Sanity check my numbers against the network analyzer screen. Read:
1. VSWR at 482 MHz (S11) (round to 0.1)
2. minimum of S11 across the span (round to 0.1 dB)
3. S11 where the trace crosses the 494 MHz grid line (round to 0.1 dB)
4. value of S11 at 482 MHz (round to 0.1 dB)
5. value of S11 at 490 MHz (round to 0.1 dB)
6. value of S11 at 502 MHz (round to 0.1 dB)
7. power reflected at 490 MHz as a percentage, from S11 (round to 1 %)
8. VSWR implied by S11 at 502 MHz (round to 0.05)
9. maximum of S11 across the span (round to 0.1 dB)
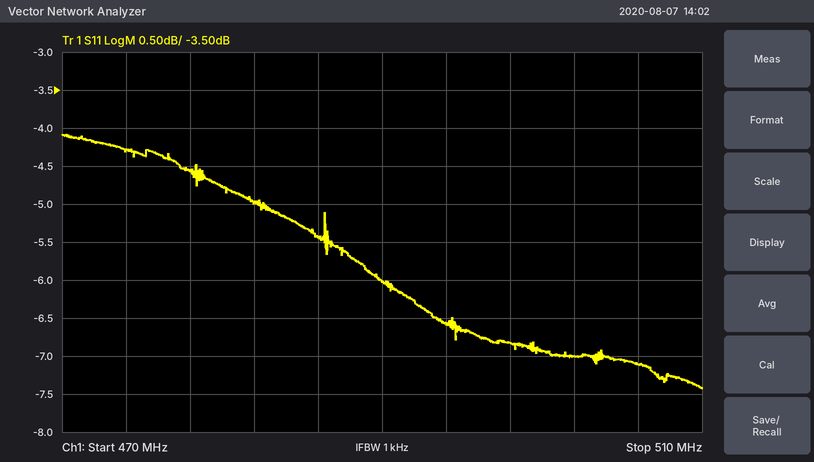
3.6
-7.4 dB
-6.6 dB
-5.0 dB
-6.0 dB
-7.0 dB
25 %
2.60
-4.1 dB
